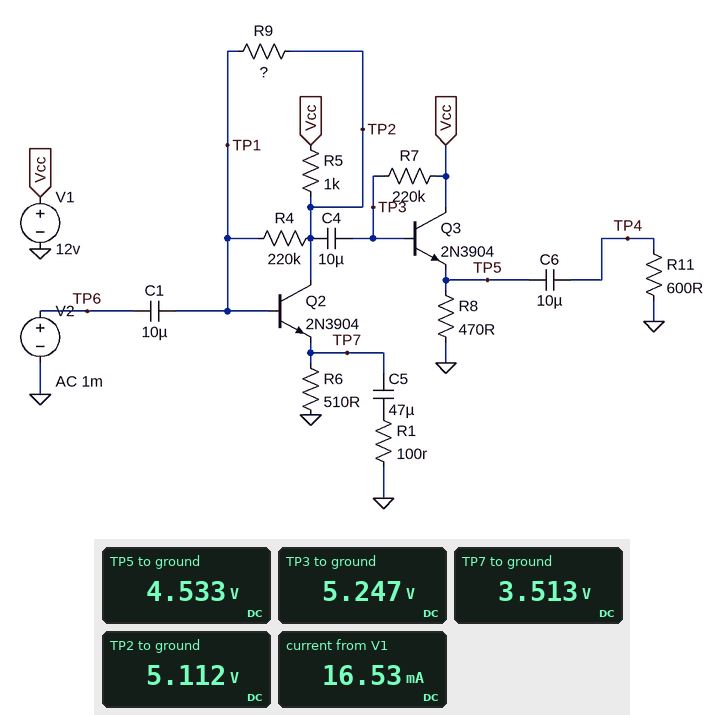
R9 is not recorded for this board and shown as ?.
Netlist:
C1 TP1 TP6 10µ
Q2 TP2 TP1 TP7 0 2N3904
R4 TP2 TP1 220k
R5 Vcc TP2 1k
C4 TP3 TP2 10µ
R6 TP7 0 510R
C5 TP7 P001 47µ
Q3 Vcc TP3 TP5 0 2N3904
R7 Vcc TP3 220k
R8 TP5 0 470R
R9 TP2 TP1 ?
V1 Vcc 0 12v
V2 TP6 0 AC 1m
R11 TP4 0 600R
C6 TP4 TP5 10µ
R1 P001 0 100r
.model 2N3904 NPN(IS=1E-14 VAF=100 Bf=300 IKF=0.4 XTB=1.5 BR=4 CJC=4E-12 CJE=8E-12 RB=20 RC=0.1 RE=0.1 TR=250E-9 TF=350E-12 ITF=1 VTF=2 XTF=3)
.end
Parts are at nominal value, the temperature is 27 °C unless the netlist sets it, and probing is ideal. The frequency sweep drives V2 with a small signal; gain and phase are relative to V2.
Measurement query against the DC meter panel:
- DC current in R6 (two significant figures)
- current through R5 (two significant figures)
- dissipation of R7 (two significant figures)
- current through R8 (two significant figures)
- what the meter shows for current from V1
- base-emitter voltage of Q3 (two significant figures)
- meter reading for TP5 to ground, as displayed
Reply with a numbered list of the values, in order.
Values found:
1. 6.9 mA
2. 6.9 mA
3. 210 µW
4. 9.6 mA
5. 16.53 mA
6. 710 mV
7. 4.533 V
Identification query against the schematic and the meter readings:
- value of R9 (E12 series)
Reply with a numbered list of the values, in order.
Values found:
1. 47 kΩ
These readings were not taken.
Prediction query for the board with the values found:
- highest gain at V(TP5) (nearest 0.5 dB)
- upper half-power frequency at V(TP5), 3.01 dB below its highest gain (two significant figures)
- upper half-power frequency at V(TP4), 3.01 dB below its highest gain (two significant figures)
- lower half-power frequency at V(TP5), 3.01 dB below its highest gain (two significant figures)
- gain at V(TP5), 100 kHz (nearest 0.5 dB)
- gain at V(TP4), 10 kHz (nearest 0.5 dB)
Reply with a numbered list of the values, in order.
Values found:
1. 20.5 dB
2. 23 MHz
3. 23 MHz
4. 36 Hz
5. 20.5 dB
6. 20.5 dB
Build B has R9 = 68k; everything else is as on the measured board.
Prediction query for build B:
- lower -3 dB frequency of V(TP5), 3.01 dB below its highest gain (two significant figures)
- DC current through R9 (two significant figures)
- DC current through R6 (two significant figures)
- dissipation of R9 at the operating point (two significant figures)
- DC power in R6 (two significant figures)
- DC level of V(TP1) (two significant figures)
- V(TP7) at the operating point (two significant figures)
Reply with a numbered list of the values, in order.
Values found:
1. 35 Hz
2. 17 µA
3. 6.7 mA
4. 20 µW
5. 23 mW
6. 4.1 V
7. 3.4 V
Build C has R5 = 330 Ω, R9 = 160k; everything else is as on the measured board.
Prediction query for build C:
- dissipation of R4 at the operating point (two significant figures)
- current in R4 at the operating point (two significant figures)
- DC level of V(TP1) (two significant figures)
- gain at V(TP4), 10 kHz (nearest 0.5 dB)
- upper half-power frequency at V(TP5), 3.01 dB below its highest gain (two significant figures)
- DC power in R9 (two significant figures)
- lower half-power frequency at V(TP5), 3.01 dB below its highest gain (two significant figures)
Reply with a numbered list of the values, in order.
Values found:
1. 41 µW
2. 14 µA
3. 5.7 V
4. 11.5 dB
5. 72 MHz
6. 57 µW
7. 33 Hz
